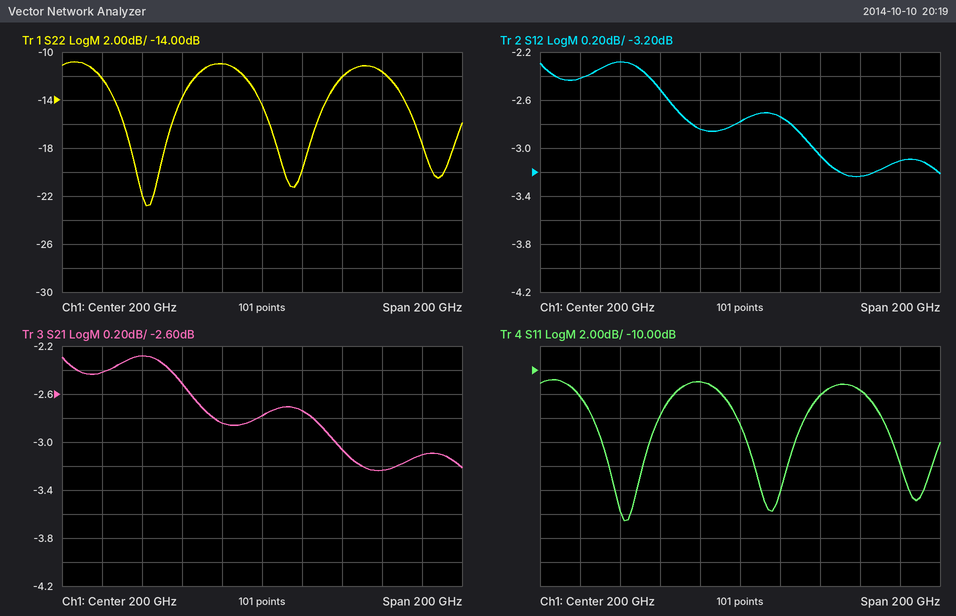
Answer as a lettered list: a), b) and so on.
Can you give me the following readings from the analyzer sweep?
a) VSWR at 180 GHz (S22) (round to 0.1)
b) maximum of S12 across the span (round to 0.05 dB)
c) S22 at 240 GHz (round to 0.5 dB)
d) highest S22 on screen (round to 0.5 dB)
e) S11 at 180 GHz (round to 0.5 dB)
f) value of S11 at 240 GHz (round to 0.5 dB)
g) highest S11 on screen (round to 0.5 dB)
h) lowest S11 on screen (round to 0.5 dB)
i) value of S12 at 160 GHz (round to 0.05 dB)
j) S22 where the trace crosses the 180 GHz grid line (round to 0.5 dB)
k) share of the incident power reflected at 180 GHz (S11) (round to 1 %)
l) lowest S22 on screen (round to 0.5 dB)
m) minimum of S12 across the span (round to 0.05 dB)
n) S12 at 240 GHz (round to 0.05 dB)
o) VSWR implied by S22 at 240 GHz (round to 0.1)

a) 1.8
b) -2.30 dB
c) -12.0 dB
d) -11.0 dB
e) -11.0 dB
f) -12.0 dB
g) -11.0 dB
h) -22.5 dB
i) -2.50 dB
j) -11.0 dB
k) 8 %
l) -23.0 dB
m) -3.25 dB
n) -3.05 dB
o) 1.7
